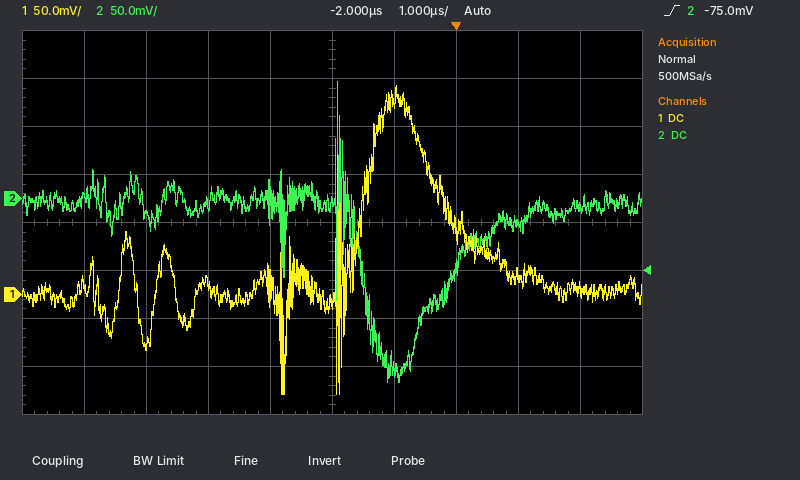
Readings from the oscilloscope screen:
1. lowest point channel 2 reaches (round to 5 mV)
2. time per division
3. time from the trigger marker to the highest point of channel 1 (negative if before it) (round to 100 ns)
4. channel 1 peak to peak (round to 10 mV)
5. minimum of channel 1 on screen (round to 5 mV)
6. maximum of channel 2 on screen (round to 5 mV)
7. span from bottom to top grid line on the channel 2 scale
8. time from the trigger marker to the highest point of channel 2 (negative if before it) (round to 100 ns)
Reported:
-190 mV
1 µs
-1.0 µs
320 mV
-105 mV
120 mV
400 mV
-1.9 µs
